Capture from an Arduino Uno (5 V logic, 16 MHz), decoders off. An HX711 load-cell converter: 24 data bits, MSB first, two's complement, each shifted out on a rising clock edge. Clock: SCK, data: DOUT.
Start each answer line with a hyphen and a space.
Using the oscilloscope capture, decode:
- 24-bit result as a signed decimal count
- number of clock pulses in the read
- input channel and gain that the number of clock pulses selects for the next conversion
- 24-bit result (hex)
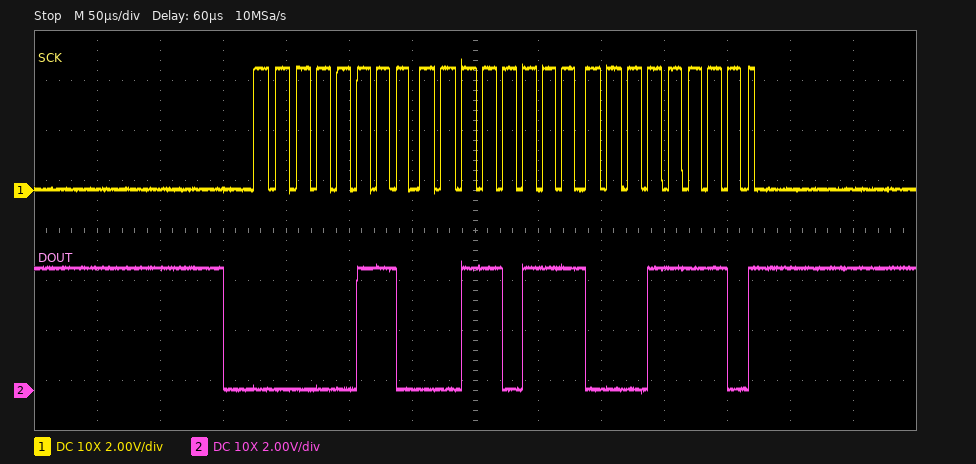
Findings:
- 407326
- 25
- channel A, gain 128
- 0x06371E
